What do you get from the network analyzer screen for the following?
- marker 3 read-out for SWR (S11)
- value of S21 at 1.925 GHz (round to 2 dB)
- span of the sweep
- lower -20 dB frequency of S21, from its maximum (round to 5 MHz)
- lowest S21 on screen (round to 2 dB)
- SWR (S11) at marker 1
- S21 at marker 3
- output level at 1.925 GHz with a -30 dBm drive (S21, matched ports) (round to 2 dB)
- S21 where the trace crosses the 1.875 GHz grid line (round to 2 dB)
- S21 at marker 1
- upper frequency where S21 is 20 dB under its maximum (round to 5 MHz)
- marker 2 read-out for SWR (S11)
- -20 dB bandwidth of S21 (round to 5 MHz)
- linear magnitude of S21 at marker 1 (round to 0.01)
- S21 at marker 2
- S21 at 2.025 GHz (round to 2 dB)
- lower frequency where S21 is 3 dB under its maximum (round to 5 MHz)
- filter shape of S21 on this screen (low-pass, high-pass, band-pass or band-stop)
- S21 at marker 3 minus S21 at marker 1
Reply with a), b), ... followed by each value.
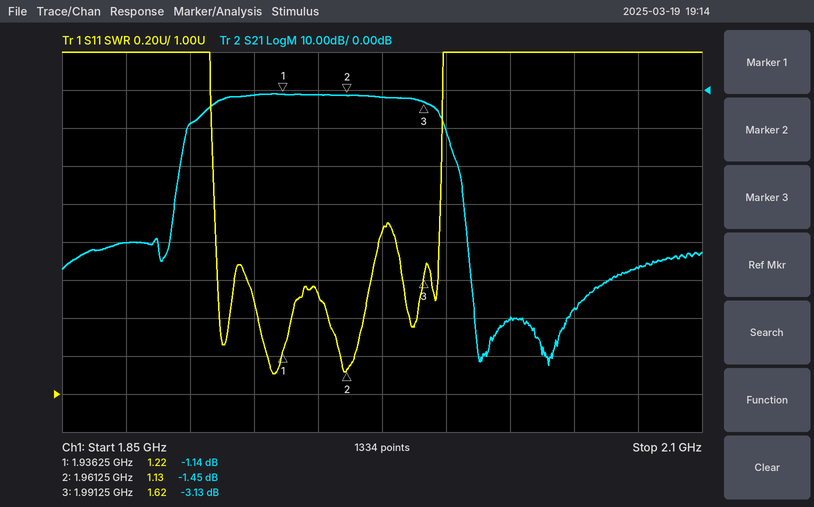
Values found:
a) 1.62
b) -2 dB
c) 250 MHz
d) 1.895 GHz
e) -72 dB
f) 1.22
g) -3.13 dB
h) -32 dBm
i) -40 dB
j) -1.14 dB
k) 2.005 GHz
l) 1.13
m) 110 MHz
n) 0.88
o) -1.45 dB
p) -60 dB
q) 1.910 GHz
r) band-pass
s) -1.99 dB
